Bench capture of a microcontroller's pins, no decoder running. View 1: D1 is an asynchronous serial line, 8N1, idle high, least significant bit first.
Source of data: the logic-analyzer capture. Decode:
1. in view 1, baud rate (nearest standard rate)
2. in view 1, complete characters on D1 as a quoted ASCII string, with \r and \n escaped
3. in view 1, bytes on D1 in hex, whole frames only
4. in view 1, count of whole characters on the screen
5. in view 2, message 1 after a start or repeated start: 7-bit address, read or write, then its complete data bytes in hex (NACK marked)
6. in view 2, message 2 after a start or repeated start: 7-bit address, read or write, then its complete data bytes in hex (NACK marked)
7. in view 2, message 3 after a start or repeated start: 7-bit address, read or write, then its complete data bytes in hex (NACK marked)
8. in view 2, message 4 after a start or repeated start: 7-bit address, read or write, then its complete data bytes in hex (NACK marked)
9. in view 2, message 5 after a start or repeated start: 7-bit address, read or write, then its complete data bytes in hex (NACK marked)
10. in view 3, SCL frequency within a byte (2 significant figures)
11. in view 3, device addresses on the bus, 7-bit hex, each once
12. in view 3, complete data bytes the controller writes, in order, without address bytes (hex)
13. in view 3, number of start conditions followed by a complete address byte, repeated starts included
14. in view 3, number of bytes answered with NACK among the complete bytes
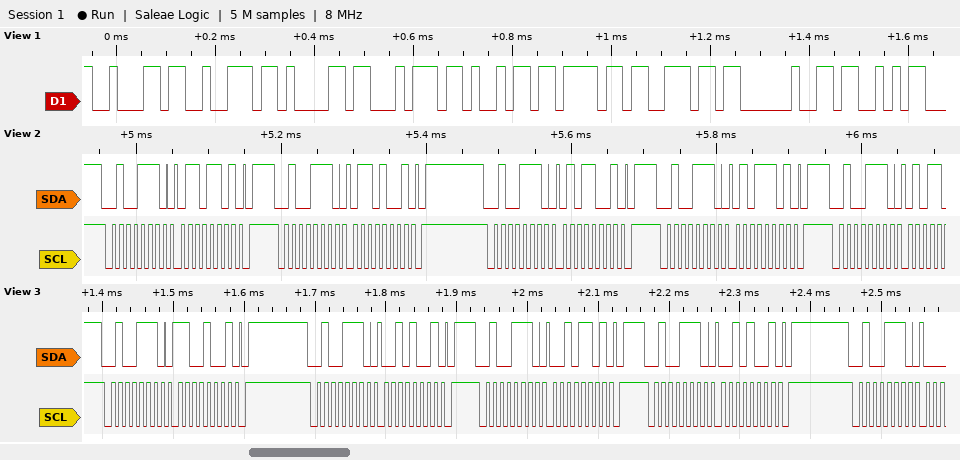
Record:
57600 baud
"bration S"
62 72 61 74 69 6F 6E 20 53
9
0x27 write: 6D
0x27 write: 69
0x27 write: 59
0x27 write: 5D
0x27 write
100 kHz
0x27
C9 29 2D 29
5
0
